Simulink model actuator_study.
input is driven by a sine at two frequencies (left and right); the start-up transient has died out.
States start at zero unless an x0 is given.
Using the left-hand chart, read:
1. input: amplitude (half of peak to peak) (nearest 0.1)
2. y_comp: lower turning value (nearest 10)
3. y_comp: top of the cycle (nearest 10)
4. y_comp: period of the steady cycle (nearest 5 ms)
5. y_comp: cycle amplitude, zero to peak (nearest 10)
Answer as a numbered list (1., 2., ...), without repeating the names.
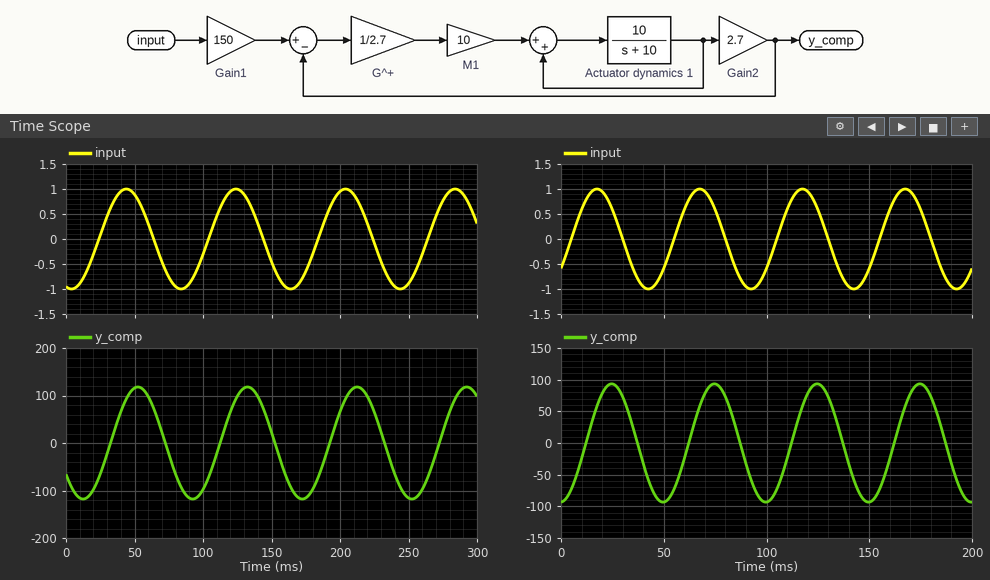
1. 1.0
2. -120
3. 120
4. 80 ms
5. 120
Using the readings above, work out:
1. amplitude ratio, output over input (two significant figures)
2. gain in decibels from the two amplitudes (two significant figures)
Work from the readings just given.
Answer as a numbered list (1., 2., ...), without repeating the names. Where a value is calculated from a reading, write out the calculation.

1. 120 / 1 = 120
2. 20 log10(120 / 1) = 42 dB
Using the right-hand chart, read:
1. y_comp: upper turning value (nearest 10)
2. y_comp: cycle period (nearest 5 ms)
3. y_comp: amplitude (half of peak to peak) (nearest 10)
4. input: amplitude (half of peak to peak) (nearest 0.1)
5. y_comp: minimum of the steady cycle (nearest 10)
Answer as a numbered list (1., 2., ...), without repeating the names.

1. 90
2. 50 ms
3. 90
4. 1.0
5. -90
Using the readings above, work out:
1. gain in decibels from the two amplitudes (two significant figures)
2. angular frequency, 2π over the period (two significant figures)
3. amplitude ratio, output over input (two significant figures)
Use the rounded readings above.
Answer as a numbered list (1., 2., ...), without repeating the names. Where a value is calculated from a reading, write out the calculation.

1. 20 log10(90 / 1) = 39 dB
2. 2π / 50 = 0.13 rad/ms
3. 90 / 1 = 90
